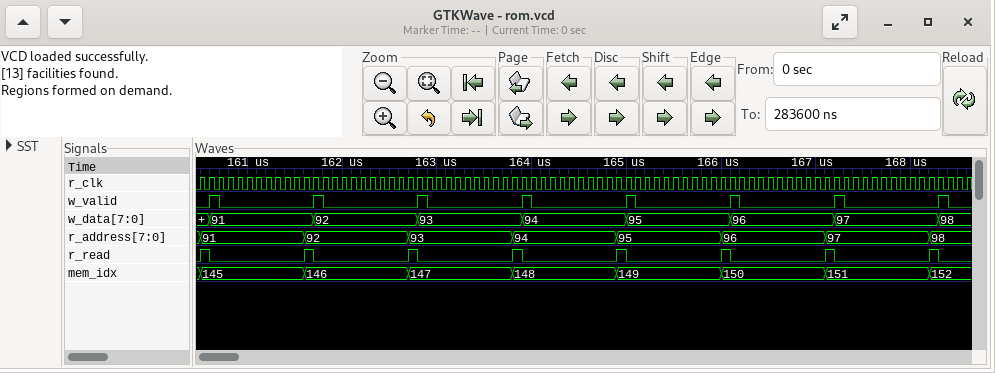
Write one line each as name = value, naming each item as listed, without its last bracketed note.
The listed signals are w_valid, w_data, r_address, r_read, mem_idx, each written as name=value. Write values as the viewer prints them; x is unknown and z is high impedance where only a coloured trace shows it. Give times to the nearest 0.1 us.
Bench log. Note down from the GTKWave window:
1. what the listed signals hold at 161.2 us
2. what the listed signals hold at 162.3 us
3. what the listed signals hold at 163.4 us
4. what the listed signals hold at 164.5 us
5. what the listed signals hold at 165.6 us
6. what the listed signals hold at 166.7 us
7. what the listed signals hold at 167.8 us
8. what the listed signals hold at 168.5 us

what the listed signals hold at 161.2 us = w_valid=0, w_data=91, r_address=91, r_read=0, mem_idx=145
what the listed signals hold at 162.3 us = w_valid=0, w_data=92, r_address=92, r_read=0, mem_idx=146
what the listed signals hold at 163.4 us = w_valid=0, w_data=93, r_address=93, r_read=0, mem_idx=147
what the listed signals hold at 164.5 us = w_valid=0, w_data=94, r_address=94, r_read=0, mem_idx=148
what the listed signals hold at 165.6 us = w_valid=0, w_data=95, r_address=95, r_read=0, mem_idx=149
what the listed signals hold at 166.7 us = w_valid=0, w_data=96, r_address=96, r_read=0, mem_idx=150
what the listed signals hold at 167.8 us = w_valid=0, w_data=97, r_address=97, r_read=0, mem_idx=151
what the listed signals hold at 168.5 us = w_valid=0, w_data=98, r_address=98, r_read=0, mem_idx=152
